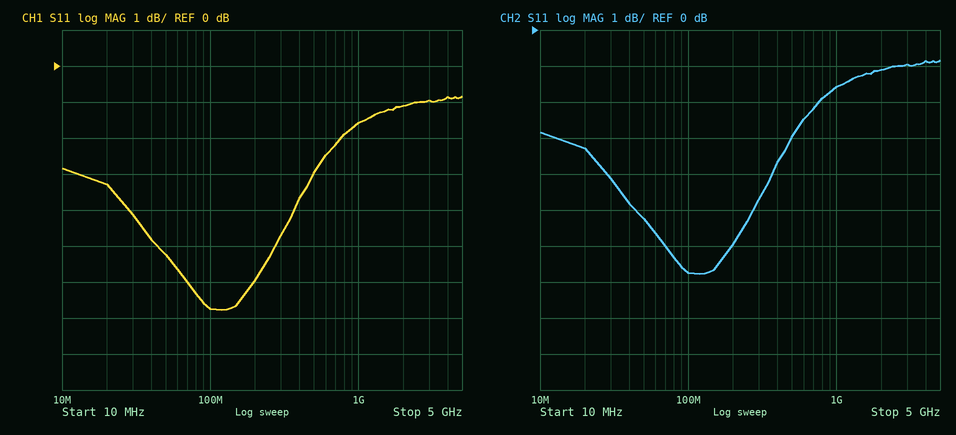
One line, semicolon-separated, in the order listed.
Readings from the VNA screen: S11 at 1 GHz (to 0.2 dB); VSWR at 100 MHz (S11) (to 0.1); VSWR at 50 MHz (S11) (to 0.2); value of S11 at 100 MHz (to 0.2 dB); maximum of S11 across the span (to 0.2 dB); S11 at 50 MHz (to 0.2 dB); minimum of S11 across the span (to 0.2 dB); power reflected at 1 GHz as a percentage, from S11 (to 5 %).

-1.6 dB; 2.7; 3.4; -6.8 dB; -0.8 dB; -5.2 dB; -6.8 dB; 70 %
